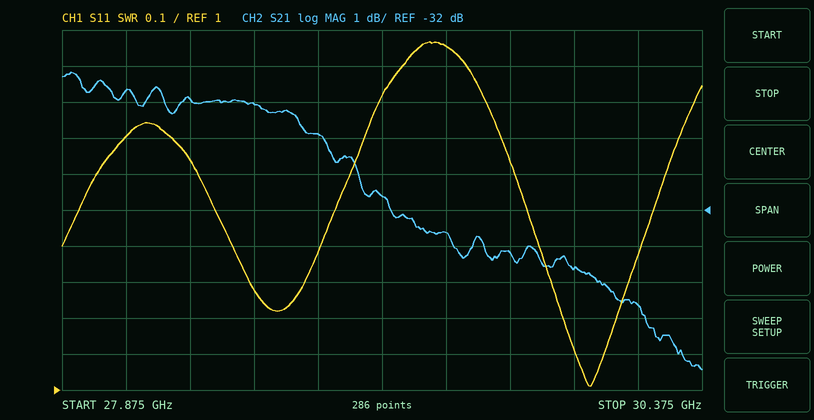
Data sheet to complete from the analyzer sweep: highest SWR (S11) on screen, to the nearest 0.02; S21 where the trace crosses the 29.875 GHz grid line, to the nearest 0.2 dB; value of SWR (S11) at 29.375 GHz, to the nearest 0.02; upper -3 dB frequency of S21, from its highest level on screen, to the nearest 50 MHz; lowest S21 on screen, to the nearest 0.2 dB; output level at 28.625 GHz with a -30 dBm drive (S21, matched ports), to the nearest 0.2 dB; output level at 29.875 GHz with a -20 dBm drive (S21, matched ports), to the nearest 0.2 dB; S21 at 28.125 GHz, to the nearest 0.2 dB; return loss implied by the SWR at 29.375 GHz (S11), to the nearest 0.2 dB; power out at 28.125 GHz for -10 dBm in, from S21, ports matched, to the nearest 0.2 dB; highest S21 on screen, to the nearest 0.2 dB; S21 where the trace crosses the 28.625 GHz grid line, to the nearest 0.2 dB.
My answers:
1.96
-33.6 dB
1.96
29.05 GHz
-36.4 dB
-59.0 dBm
-53.6 dBm
-28.6 dB
9.8 dB
-38.6 dBm
-28.2 dB
-29.0 dB
